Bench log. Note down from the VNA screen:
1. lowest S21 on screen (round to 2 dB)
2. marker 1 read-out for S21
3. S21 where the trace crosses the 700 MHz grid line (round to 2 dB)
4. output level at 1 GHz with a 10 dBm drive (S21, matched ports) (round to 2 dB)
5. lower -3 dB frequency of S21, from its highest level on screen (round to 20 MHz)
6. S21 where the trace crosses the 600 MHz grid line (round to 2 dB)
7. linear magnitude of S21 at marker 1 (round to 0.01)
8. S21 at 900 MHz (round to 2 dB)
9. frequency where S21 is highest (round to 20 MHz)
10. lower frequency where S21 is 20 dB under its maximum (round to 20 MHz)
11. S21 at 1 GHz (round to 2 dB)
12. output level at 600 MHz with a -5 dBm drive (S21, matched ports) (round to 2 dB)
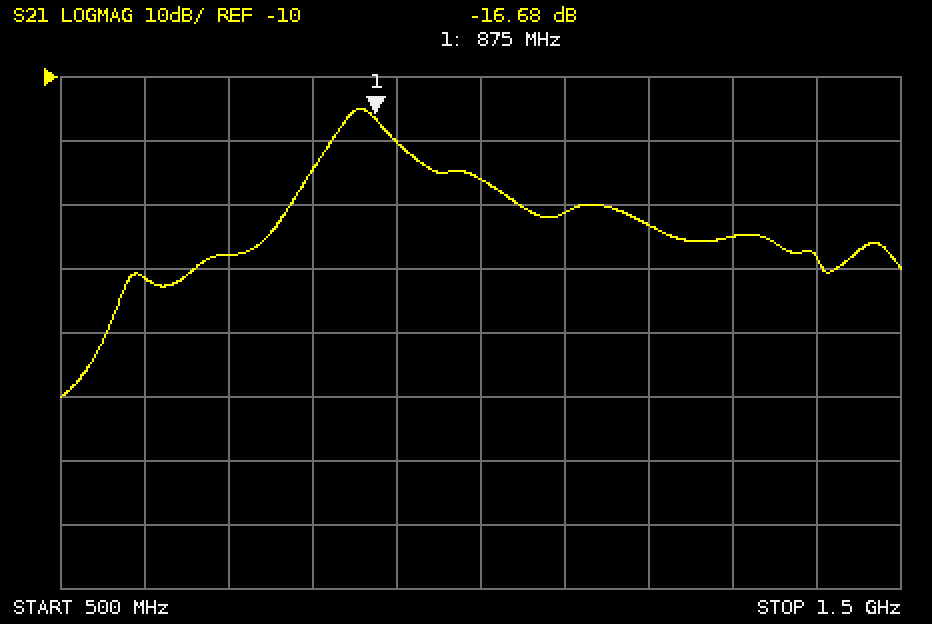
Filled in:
-60 dB
-16.68 dB
-38 dB
-16 dBm
840 MHz
-42 dB
0.15
-20 dB
860 MHz
740 MHz
-26 dB
-46 dBm
